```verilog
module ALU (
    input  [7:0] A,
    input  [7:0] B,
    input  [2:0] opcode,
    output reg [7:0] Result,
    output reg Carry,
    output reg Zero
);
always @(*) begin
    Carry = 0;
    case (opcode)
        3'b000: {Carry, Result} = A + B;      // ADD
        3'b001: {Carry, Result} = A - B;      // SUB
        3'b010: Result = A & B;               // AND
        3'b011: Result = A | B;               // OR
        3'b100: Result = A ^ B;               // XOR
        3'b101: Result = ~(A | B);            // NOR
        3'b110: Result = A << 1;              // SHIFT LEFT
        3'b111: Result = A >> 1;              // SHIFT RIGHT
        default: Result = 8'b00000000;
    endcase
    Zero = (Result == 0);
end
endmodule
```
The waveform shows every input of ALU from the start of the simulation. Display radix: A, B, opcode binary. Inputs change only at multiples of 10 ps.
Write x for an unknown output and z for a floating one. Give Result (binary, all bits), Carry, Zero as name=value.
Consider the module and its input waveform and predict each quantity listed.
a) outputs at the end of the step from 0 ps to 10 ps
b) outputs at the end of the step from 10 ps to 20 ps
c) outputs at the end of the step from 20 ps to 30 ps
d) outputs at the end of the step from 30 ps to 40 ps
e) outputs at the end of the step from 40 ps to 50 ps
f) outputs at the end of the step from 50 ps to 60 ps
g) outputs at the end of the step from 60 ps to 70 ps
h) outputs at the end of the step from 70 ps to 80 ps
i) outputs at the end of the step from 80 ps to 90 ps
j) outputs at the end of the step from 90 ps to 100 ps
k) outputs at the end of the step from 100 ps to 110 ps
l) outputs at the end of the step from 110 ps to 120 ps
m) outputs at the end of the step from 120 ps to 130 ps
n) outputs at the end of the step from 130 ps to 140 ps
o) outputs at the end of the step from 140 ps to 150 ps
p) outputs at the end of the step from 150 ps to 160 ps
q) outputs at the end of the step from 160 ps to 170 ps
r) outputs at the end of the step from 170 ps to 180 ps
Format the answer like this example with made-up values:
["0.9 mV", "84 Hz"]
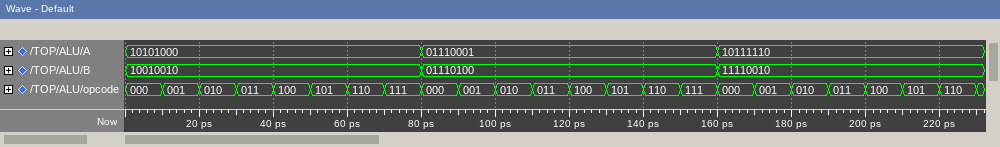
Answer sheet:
["Result=00111010, Carry=1, Zero=0", "Result=00010110, Carry=0, Zero=0", "Result=10000000, Carry=0, Zero=0", "Result=10111010, Carry=0, Zero=0", "Result=00111010, Carry=0, Zero=0", "Result=01000101, Carry=0, Zero=0", "Result=01010000, Carry=0, Zero=0", "Result=01010100, Carry=0, Zero=0", "Result=11100101, Carry=0, Zero=0", "Result=11111101, Carry=1, Zero=0", "Result=01110000, Carry=0, Zero=0", "Result=01110101, Carry=0, Zero=0", "Result=00000101, Carry=0, Zero=0", "Result=10001010, Carry=0, Zero=0", "Result=11100010, Carry=0, Zero=0", "Result=00111000, Carry=0, Zero=0", "Result=10110000, Carry=1, Zero=0", "Result=11001100, Carry=1, Zero=0"]
